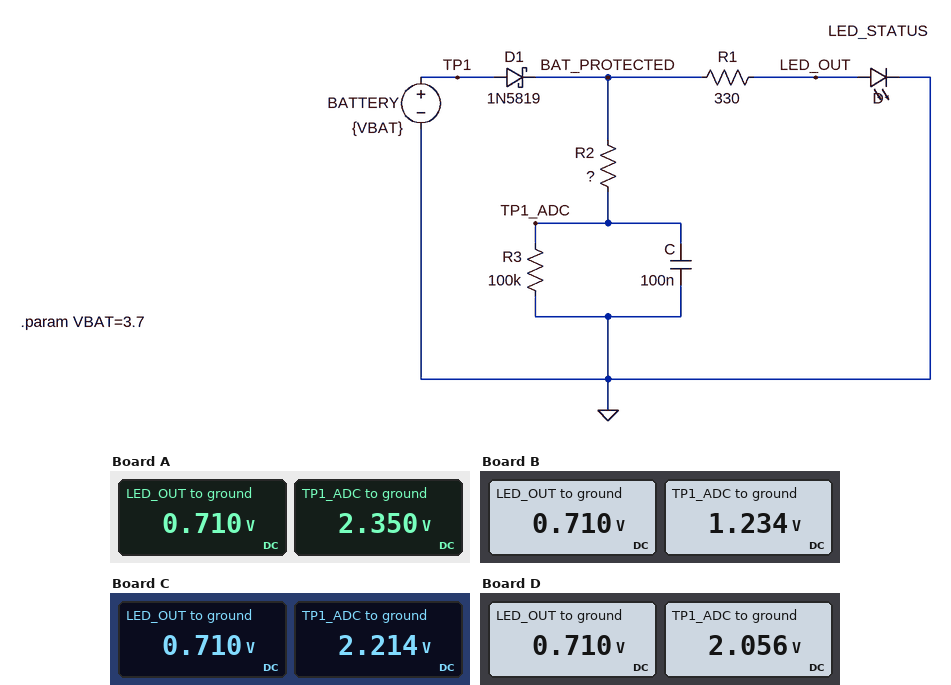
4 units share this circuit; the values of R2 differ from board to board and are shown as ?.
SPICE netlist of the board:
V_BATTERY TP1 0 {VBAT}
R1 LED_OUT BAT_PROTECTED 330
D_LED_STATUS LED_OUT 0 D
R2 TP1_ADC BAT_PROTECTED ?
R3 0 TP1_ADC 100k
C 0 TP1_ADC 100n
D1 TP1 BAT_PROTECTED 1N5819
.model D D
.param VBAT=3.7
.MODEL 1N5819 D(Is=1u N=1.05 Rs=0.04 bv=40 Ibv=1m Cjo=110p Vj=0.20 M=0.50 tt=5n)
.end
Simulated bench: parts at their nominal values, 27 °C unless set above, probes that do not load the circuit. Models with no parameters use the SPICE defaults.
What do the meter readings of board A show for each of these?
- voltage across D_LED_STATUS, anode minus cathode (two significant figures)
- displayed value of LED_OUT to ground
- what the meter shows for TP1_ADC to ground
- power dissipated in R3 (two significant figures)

710 mV
0.710 V
2.350 V
55 µW
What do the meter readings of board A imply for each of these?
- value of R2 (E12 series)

47 kΩ
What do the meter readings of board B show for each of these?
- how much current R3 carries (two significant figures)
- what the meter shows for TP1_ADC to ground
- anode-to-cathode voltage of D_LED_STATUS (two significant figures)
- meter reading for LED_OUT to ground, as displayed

12 µA
1.234 V
710 mV
0.710 V
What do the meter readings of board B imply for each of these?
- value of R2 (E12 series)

180 kΩ
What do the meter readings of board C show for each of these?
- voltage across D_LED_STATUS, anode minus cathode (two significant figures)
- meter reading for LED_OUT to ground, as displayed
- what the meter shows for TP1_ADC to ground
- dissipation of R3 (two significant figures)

710 mV
0.710 V
2.214 V
49 µW
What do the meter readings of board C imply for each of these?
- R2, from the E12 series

56 kΩ
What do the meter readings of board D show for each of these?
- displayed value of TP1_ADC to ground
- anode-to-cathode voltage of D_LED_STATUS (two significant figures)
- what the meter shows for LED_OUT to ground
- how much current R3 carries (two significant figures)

2.056 V
710 mV
0.710 V
21 µA
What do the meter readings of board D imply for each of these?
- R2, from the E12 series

68 kΩ
